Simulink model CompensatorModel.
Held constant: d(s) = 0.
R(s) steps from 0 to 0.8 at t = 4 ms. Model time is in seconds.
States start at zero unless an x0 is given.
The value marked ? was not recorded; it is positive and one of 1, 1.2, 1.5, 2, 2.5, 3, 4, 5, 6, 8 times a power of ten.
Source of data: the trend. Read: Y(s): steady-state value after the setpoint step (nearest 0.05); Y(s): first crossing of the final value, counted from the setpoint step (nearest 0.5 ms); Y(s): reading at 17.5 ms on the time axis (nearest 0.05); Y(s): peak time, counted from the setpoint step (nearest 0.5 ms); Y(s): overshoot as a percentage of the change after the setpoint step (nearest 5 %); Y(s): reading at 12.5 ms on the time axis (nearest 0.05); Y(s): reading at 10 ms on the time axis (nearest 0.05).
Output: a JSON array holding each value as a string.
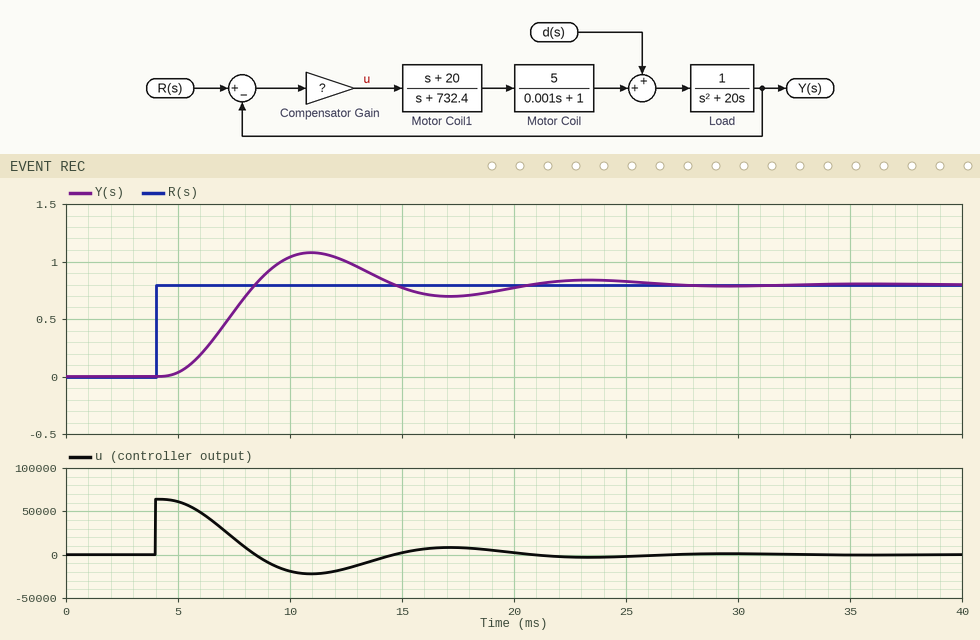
["0.80", "4.5 ms", "0.70", "7.0 ms", "35 %", "1.00", "1.05"]
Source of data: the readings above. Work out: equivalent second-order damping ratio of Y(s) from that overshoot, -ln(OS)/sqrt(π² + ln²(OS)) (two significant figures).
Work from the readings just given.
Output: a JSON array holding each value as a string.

["0.32"]
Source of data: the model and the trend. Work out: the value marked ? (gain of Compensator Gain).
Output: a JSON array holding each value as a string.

["80000"]
